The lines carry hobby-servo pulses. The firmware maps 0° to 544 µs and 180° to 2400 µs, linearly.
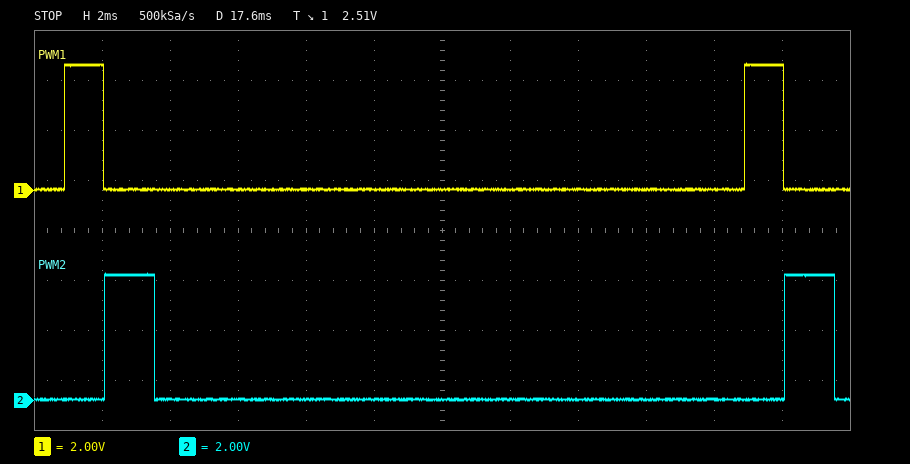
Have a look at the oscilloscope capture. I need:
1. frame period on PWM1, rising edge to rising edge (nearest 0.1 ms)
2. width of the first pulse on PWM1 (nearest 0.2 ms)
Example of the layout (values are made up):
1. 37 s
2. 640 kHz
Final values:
1. 20.0 ms
2. 1.2 ms
